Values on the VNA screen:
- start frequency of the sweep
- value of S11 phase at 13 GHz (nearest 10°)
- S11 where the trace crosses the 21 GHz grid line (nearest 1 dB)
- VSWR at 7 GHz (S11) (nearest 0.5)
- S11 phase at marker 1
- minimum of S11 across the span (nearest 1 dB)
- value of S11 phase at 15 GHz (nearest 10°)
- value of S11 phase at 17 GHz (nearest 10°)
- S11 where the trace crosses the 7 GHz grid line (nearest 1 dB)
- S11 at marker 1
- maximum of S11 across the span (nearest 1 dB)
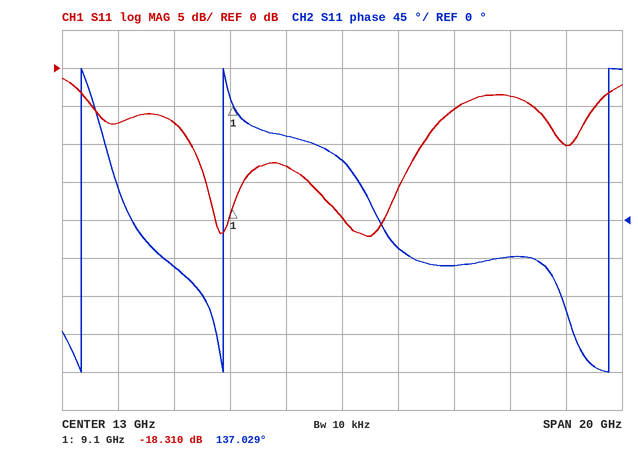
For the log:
3 GHz
70°
-10 dB
2.5
137.029°
-22 dB
-30°
-50°
-7 dB
-18.310 dB
-1 dB
